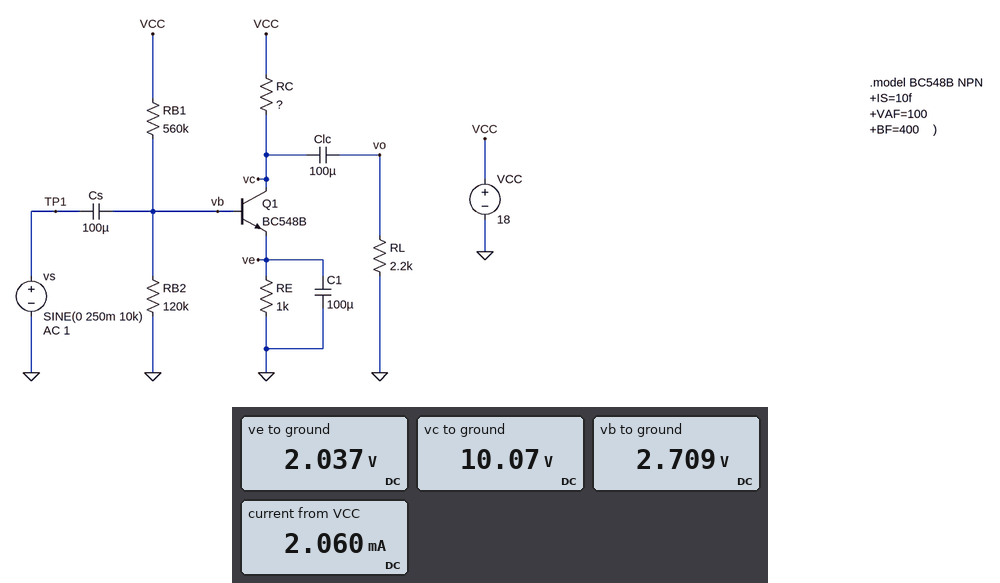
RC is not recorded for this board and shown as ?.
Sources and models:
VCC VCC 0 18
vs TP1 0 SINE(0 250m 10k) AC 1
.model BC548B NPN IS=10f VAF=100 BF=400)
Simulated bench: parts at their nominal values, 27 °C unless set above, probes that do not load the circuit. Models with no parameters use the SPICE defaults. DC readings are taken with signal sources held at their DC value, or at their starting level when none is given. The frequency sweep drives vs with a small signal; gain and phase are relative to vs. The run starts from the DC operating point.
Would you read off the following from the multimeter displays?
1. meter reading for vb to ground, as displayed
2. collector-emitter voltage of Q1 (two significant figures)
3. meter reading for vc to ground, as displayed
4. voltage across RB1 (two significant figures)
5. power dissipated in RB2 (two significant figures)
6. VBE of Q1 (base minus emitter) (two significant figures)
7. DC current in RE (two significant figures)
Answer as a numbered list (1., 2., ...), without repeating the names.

1. 2.709 V
2. 8.0 V
3. 10.07 V
4. 15 V
5. 61 µW
6. 670 mV
7. 2.0 mA
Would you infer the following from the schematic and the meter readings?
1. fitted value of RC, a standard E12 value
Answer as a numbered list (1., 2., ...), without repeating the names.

1. 3.9 kΩ
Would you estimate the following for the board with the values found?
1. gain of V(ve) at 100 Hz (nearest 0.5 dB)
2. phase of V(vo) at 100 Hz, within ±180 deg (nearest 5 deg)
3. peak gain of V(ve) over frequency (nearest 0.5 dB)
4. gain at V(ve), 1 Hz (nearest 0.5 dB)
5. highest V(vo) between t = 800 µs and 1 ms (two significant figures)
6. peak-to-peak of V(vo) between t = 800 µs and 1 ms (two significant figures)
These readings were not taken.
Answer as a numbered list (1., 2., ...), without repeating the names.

1. -2.5 dB
2. -130 deg
3. 0 dB
4. 0 dB
5. 2.9 V
6. 11 V
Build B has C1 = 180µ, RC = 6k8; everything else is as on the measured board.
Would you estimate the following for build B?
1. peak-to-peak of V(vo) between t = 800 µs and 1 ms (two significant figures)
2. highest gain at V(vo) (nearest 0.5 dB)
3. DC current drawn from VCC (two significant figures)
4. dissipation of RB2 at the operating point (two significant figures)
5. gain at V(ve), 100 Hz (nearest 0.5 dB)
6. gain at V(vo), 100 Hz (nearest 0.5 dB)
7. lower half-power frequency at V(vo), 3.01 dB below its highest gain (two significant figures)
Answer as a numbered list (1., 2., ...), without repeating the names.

1. 5.6 V
2. 42.0 dB
3. 2.0 mA
4. 60 µW
5. -5.0 dB
6. 40.5 dB
7. 68 Hz
